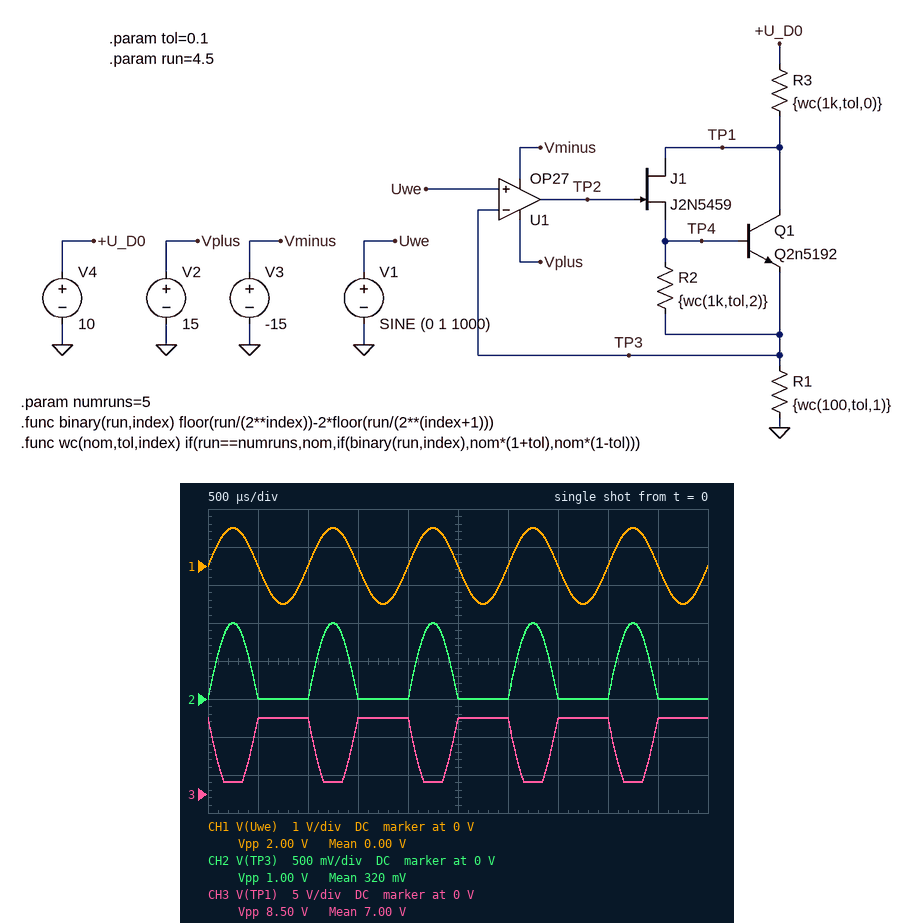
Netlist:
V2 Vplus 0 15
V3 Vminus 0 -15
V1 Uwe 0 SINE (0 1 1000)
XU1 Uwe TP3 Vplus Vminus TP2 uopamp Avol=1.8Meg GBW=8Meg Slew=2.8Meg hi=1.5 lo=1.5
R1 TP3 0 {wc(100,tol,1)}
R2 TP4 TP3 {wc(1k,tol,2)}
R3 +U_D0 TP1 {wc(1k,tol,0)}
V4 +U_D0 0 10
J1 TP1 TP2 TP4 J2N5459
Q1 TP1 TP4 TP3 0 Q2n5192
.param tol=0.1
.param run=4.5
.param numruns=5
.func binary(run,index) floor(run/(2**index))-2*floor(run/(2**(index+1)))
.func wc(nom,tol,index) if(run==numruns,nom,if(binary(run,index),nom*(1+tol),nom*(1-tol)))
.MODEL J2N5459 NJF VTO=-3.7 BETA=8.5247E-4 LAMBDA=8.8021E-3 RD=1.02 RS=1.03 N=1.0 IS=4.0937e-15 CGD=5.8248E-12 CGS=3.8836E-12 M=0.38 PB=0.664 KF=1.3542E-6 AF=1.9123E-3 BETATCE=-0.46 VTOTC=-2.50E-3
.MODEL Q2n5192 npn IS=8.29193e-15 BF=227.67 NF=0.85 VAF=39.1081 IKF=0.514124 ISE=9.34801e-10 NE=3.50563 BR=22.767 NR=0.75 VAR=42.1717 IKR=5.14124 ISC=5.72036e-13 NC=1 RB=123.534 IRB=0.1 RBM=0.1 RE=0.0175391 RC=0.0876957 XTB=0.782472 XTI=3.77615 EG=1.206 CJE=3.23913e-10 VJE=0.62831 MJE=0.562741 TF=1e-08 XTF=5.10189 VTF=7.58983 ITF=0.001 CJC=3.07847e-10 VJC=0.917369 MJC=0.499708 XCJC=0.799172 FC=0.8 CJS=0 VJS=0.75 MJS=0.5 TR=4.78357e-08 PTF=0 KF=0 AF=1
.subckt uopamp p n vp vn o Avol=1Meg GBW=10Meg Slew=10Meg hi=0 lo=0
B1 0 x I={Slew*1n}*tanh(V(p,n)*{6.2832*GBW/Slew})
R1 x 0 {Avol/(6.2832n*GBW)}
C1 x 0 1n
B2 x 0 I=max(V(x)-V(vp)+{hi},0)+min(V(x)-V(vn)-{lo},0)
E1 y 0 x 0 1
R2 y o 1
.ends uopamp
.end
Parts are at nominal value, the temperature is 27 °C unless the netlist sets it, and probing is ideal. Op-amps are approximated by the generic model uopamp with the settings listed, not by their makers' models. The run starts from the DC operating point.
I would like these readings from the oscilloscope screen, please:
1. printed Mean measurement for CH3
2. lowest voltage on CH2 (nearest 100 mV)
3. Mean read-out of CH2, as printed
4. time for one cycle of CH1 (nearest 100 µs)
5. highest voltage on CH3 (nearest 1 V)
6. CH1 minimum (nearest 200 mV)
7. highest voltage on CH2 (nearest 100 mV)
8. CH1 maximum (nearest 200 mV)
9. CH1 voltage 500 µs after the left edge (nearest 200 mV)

7.00 V
0 V
320 mV
1.0 ms
10 V
-1.0 V
1.0 V
1.0 V
0 V
